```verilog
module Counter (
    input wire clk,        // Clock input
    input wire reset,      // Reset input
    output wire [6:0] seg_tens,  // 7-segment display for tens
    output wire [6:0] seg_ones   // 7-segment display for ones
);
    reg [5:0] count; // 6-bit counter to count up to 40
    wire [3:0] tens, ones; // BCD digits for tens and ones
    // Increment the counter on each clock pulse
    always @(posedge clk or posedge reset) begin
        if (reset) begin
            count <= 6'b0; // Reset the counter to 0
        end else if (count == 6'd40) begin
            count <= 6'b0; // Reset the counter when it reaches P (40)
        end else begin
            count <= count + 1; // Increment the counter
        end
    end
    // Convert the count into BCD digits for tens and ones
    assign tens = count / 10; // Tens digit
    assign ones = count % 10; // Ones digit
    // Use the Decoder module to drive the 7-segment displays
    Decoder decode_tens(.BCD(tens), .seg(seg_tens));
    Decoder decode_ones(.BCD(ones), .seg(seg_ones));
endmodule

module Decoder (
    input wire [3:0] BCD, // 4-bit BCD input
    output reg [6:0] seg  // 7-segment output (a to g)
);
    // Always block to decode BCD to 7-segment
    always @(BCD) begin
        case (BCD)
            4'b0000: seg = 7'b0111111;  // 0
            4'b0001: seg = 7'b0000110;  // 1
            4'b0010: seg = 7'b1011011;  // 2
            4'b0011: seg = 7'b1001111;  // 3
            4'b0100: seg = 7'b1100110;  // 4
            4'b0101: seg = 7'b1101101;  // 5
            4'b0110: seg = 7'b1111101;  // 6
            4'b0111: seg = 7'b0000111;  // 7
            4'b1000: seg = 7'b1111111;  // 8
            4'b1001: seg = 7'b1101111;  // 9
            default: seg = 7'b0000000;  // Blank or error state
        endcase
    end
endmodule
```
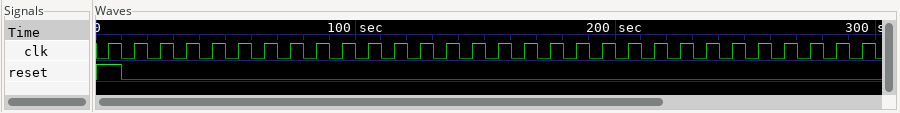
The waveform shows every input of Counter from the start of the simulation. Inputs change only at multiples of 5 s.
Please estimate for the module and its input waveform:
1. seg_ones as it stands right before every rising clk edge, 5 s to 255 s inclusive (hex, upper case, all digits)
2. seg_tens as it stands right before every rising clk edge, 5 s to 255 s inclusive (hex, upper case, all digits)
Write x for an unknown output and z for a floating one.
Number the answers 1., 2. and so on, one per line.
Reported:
1. 3F, 3F, 06, 5B, 4F, 66, 6D, 7D, 07, 7F, 6F, 3F, 06, 5B, 4F, 66, 6D, 7D, 07, 7F, 6F, 3F, 06, 5B, 4F, 66
2. 3F, 3F, 3F, 3F, 3F, 3F, 3F, 3F, 3F, 3F, 3F, 06, 06, 06, 06, 06, 06, 06, 06, 06, 06, 5B, 5B, 5B, 5B, 5B
